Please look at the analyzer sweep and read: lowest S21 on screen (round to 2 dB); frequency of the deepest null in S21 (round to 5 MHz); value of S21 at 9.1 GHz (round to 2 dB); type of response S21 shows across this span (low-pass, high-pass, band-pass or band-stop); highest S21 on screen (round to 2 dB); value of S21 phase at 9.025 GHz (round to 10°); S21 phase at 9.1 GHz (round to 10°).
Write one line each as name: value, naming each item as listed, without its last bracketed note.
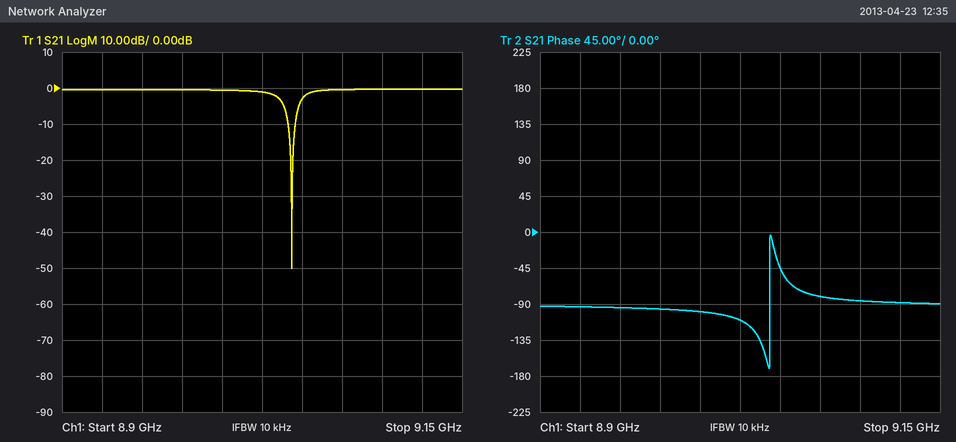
lowest S21 on screen: -50 dB
frequency of the deepest null in S21: 9.045 GHz
value of S21 at 9.1 GHz: 0 dB
type of response S21 shows across this span: band-stop
highest S21 on screen: 0 dB
value of S21 phase at 9.025 GHz: -110°
S21 phase at 9.1 GHz: -90°
